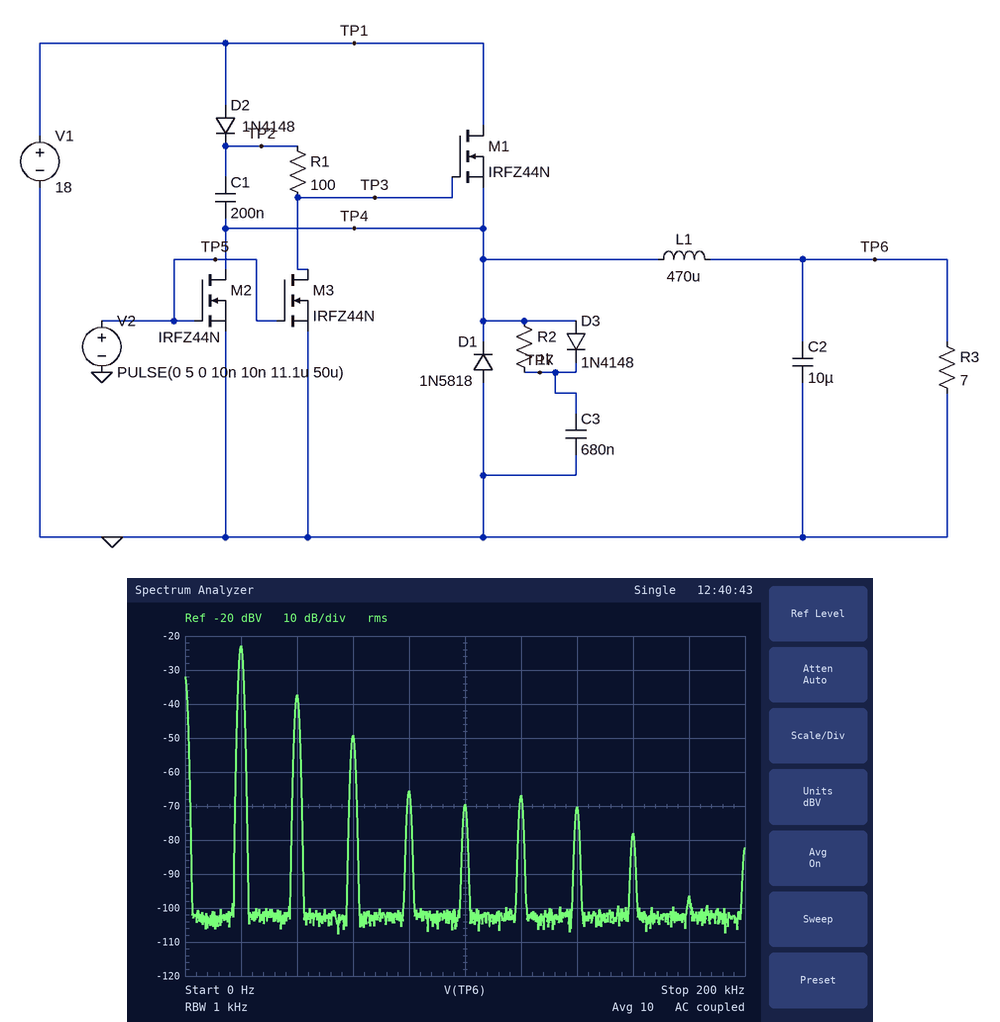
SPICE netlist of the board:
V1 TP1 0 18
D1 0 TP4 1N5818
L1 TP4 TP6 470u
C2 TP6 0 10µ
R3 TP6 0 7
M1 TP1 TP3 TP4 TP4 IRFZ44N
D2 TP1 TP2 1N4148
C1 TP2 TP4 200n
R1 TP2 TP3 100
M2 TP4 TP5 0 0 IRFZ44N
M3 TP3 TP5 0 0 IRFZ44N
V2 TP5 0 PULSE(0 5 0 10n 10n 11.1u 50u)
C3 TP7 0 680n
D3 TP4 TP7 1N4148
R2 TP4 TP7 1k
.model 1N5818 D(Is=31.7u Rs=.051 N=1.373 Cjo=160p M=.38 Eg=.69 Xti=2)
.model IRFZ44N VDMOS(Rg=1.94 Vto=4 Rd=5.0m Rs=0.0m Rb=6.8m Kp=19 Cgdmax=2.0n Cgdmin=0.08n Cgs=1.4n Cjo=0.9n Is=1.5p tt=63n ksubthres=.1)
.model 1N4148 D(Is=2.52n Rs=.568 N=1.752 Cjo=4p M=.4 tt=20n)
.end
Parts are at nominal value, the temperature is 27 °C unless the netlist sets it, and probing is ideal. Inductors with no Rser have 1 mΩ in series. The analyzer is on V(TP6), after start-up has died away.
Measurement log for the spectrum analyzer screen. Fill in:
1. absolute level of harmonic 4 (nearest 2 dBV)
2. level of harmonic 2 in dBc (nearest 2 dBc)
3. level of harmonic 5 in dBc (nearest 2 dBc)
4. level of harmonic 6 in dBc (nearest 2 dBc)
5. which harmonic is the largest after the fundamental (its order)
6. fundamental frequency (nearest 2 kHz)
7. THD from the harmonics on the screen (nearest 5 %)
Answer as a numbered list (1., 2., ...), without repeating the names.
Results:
1. -66 dBV
2. -14 dBc
3. -46 dBc
4. -44 dBc
5. 2
6. 20 kHz
7. 20 %
